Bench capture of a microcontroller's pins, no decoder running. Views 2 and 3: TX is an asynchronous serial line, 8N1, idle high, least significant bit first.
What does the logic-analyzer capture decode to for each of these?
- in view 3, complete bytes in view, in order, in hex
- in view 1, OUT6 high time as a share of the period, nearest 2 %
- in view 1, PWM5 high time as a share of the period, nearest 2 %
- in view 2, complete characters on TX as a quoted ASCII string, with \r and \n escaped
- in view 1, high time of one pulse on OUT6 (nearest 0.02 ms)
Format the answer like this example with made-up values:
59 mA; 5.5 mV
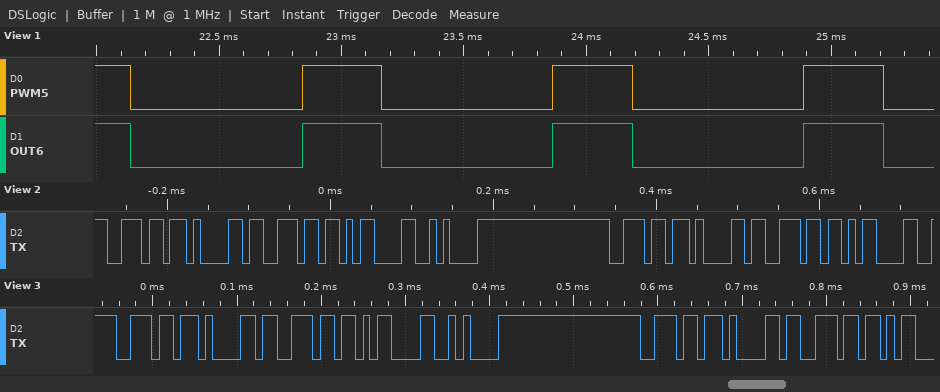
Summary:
6E 61 6E 0D 0A 6E 61 6E; 32 %; 32 %; "nan\r\nnan\r"; 0.32 ms
